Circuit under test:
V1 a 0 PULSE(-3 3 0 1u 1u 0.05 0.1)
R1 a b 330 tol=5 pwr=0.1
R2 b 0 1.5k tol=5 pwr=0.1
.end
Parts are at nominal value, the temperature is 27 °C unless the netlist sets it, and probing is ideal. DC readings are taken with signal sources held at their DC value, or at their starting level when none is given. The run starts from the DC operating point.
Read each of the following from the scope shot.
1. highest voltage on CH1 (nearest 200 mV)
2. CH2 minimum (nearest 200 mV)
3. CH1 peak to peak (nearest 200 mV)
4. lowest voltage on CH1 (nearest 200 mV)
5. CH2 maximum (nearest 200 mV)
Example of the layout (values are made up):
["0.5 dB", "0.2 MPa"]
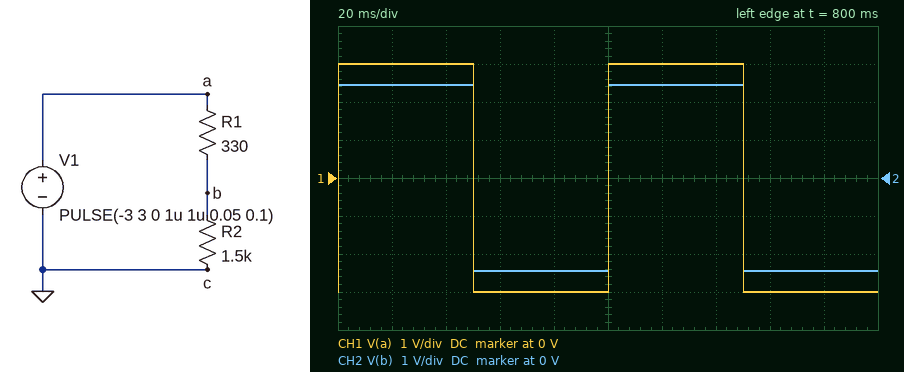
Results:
["3.0 V", "-2.4 V", "6.0 V", "-3.0 V", "2.4 V"]
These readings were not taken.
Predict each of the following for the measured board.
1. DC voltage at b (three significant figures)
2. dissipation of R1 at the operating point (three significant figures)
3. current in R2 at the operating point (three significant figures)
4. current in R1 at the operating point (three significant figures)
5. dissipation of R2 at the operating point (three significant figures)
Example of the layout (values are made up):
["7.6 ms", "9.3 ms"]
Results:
["-2.46 V", "887 µW", "1.64 mA", "1.64 mA", "4.03 mW"]
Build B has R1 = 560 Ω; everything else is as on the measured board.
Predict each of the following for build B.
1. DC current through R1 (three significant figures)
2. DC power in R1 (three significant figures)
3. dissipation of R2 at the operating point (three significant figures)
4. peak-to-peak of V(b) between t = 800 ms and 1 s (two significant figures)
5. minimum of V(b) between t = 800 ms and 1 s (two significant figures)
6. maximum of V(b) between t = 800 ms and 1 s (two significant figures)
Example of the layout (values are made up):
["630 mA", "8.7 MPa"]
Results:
["1.46 mA", "1.19 mW", "3.18 mW", "4.4 V", "-2.2 V", "2.2 V"]
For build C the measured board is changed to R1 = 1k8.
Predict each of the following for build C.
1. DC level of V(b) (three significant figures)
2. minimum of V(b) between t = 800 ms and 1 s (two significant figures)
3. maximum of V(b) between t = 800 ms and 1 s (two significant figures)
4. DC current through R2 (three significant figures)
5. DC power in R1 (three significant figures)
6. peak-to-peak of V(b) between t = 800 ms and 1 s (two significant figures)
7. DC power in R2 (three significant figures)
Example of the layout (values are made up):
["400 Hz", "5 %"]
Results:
["-1.36 V", "-1.4 V", "1.4 V", "909 µA", "1.49 mW", "2.7 V", "1.24 mW"]
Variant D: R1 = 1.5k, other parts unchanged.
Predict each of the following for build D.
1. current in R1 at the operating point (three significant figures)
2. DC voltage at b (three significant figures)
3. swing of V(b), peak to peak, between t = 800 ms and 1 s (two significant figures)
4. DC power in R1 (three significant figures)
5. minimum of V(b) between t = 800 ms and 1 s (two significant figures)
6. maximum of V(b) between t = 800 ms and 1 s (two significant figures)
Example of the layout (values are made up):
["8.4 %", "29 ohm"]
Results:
["1.00 mA", "-1.50 V", "3.0 V", "1.50 mW", "-1.5 V", "1.5 V"]
